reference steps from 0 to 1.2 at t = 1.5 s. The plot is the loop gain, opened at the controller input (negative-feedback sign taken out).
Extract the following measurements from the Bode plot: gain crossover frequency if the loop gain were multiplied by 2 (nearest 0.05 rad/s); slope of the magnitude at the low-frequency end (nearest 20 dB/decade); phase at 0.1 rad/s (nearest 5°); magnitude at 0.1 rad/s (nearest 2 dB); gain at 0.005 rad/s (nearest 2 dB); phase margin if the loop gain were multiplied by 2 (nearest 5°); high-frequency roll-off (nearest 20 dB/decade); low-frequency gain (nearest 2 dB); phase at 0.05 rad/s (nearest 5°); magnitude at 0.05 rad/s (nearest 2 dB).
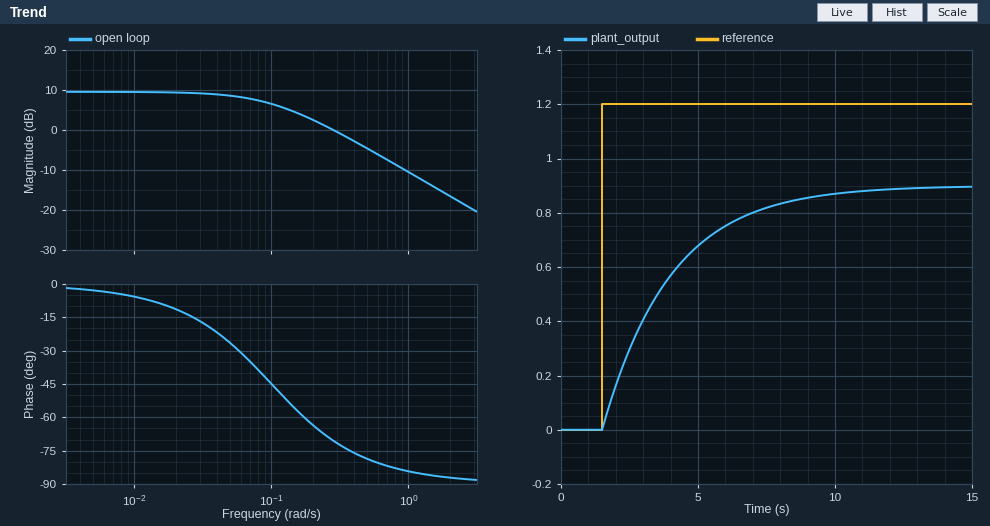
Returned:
0.60 rad/s
0 dB/decade
-45°
6 dB
10 dB
100°
-20 dB/decade
10 dB
-25°
8 dB
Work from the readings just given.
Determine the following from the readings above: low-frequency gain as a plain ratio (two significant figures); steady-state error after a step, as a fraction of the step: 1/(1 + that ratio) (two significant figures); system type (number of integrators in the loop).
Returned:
3.2
0.24
0
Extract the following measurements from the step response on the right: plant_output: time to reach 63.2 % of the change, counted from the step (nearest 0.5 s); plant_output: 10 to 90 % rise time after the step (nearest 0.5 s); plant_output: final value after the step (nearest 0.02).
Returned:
2.5 s
5.5 s
0.90
